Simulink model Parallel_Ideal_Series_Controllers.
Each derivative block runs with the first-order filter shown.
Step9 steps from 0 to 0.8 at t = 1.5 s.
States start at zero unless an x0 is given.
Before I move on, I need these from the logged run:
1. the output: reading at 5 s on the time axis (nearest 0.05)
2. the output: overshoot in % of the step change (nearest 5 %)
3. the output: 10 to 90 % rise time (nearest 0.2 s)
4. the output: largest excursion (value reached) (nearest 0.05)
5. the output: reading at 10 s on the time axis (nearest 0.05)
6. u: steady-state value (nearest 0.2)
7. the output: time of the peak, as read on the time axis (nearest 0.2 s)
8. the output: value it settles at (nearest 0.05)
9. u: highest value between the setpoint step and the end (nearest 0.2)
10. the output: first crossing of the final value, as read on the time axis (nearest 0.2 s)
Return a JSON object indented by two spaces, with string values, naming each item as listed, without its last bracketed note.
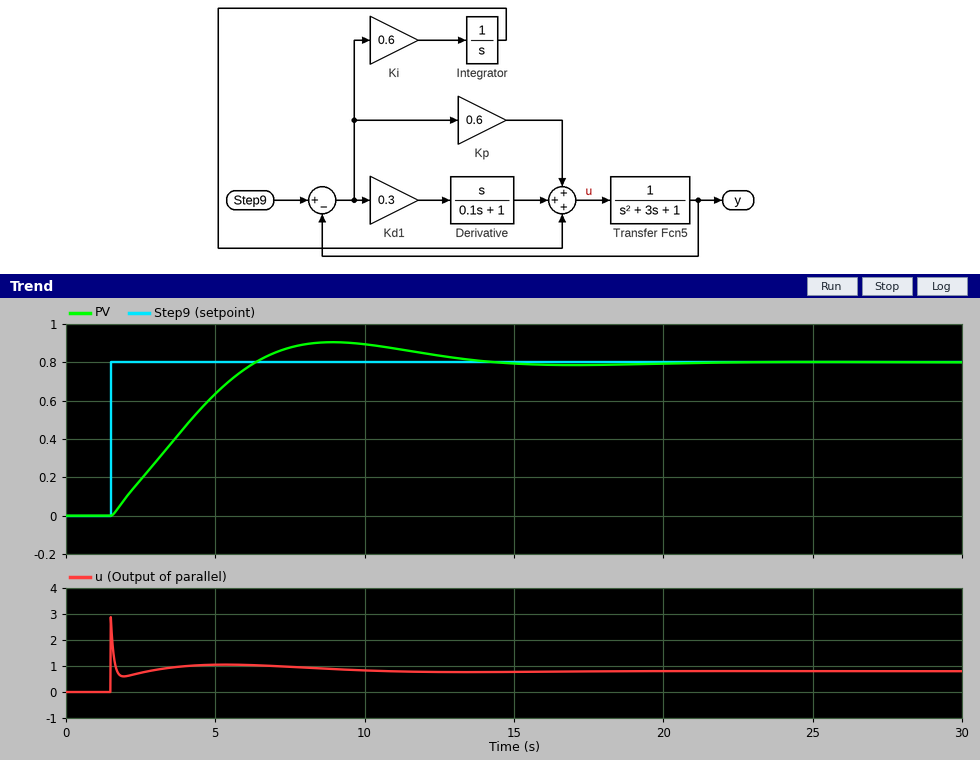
{
  "the output: reading at 5 s on the time axis": "0.65",
  "the output: overshoot in % of the step change": "15 %",
  "the output: 10 to 90 % rise time": "3.6 s",
  "the output: largest excursion (value reached)": "0.90",
  "the output: reading at 10 s on the time axis": "0.90",
  "u: steady-state value": "0.8",
  "the output: time of the peak, as read on the time axis": "9.0 s",
  "the output: value it settles at": "0.80",
  "u: highest value between the setpoint step and the end": "2.8",
  "the output: first crossing of the final value, as read on the time axis": "6.4 s"
}
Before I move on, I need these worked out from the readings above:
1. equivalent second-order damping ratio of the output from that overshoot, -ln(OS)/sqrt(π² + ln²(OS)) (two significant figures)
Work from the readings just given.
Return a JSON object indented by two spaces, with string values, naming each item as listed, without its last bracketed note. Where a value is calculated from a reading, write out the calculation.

{
  "equivalent second-order damping ratio of the output from that overshoot, -ln(OS)/sqrt(π² + ln²(OS))": "ln(0.15) = -1.897; 1.897 / sqrt(9.870 + 3.599) = 0.52"
}
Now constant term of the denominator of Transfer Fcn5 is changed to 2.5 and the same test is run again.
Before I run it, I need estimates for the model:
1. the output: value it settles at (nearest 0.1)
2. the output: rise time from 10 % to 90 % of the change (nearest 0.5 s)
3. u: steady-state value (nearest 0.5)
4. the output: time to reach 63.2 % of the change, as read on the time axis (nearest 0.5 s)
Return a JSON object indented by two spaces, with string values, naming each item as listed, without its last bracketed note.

{
  "the output: value it settles at": "0.8",
  "the output: rise time from 10 % to 90 % of the change": "9.0 s",
  "u: steady-state value": "2.0",
  "the output: time to reach 63.2 % of the change, as read on the time axis": "6.0 s"
}
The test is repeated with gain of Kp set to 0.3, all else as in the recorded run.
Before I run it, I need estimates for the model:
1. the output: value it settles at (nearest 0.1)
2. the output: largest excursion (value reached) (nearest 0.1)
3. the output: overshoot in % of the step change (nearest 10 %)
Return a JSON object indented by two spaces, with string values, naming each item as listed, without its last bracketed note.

{
  "the output: value it settles at": "0.8",
  "the output: largest excursion (value reached)": "1.0",
  "the output: overshoot in % of the step change": "20 %"
}
